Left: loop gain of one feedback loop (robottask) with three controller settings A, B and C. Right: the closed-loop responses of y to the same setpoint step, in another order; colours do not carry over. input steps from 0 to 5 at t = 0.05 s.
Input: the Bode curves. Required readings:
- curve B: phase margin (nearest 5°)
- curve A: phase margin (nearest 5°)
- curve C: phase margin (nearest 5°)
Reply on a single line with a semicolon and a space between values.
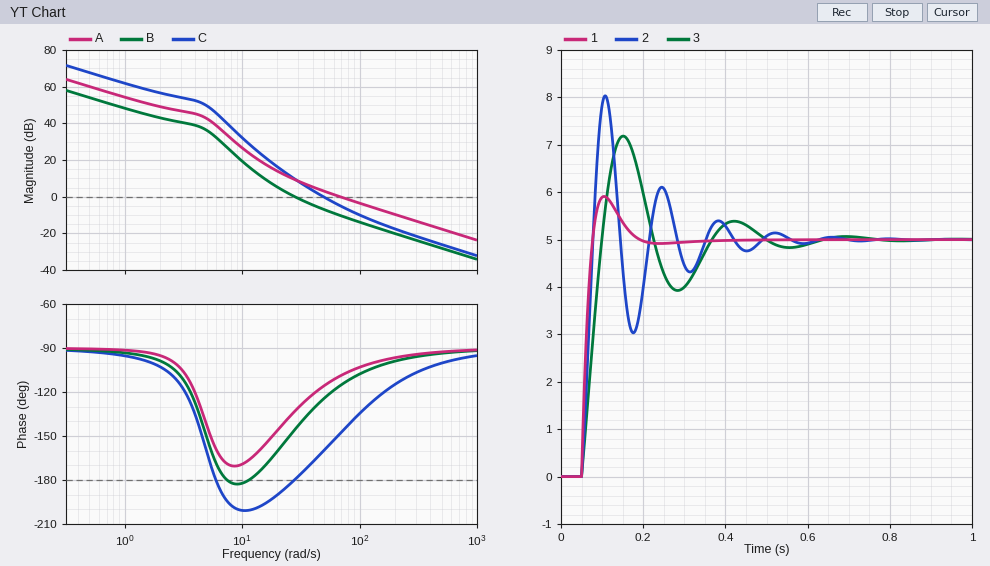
35°; 70°; 20°
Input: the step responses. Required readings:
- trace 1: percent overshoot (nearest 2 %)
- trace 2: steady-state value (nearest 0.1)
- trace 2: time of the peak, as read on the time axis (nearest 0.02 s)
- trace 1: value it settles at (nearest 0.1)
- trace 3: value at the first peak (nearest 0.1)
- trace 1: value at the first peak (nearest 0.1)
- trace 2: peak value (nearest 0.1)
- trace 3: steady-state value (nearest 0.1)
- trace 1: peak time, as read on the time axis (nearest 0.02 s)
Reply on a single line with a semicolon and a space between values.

18 %; 5.0; 0.10 s; 5.0; 7.2; 5.9; 8.0; 5.0; 0.10 s
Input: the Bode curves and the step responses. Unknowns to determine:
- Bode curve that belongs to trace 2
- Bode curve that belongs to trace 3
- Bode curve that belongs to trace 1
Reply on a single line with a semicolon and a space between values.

C; B; A
